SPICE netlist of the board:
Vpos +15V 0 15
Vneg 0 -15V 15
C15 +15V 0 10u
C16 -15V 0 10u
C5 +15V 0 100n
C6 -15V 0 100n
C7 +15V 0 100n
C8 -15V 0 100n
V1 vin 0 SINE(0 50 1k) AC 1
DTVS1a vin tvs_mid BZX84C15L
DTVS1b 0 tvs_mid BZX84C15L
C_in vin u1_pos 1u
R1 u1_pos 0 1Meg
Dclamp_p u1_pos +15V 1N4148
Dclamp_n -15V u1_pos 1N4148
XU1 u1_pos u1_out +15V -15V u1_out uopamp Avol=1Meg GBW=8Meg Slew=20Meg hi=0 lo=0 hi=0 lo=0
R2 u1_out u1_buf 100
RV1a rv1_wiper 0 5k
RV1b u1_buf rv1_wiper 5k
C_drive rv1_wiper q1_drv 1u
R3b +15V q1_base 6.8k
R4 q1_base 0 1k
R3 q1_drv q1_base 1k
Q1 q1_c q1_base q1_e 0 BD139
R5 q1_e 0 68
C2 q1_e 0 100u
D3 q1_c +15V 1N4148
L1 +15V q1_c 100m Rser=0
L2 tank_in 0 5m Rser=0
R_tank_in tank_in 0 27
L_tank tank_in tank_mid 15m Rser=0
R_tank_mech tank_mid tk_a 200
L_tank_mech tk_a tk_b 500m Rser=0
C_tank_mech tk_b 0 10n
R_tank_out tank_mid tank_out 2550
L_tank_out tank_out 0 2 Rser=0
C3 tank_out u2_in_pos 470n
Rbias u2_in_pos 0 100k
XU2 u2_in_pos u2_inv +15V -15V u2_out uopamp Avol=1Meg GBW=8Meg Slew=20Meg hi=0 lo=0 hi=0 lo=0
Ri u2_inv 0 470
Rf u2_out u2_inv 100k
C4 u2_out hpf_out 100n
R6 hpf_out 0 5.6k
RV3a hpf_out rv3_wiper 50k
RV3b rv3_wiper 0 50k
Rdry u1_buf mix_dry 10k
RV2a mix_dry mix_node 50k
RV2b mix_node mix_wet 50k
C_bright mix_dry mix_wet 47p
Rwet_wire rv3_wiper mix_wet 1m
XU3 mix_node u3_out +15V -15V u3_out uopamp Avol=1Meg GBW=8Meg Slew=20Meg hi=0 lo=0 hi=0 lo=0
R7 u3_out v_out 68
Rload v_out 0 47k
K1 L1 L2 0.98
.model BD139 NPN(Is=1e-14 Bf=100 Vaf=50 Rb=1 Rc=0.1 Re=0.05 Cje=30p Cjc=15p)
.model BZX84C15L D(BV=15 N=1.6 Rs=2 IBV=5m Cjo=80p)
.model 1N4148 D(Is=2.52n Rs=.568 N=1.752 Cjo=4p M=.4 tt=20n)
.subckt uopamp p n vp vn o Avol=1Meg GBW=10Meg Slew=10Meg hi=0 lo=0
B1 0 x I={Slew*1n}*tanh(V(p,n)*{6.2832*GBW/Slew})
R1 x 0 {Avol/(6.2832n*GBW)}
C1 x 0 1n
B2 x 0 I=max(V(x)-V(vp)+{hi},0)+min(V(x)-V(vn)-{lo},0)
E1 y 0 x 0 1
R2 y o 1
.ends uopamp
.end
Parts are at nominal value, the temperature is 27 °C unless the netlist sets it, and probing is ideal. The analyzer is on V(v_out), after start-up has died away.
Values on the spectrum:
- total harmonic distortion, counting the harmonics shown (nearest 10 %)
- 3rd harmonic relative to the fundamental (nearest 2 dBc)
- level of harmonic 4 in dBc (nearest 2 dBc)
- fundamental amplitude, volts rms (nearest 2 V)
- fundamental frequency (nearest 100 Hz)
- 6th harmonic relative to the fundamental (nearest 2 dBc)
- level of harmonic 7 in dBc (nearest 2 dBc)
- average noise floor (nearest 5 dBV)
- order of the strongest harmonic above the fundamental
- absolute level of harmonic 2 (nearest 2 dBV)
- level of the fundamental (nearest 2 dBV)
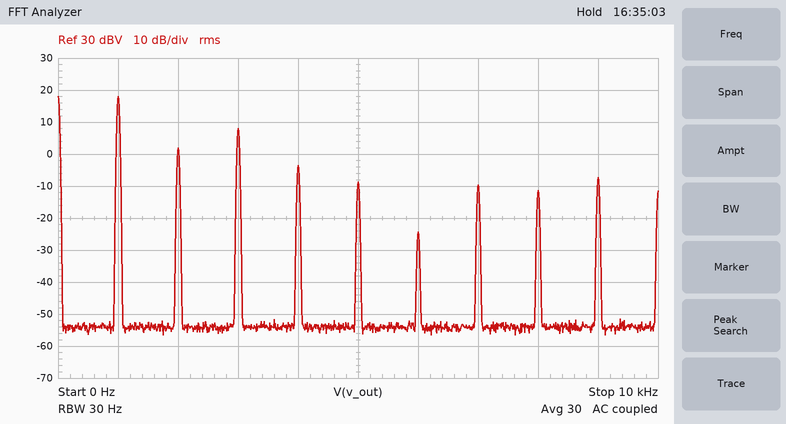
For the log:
40 %
-10 dBc
-22 dBc
8 V
1.0 kHz
-42 dBc
-28 dBc
-55 dBV
3
2 dBV
18 dBV
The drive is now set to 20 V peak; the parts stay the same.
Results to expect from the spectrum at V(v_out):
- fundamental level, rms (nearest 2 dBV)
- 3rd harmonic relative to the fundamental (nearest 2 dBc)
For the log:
18 dBV
-16 dBc
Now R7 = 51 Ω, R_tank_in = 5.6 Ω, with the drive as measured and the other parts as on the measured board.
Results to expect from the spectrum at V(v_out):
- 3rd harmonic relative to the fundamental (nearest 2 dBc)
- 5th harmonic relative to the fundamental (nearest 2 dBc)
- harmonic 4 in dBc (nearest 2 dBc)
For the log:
-14 dBc
-20 dBc
-48 dBc
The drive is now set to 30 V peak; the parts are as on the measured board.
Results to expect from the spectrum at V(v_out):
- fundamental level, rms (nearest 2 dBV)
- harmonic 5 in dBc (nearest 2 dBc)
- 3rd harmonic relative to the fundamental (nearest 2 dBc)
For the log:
18 dBV
-30 dBc
-12 dBc
